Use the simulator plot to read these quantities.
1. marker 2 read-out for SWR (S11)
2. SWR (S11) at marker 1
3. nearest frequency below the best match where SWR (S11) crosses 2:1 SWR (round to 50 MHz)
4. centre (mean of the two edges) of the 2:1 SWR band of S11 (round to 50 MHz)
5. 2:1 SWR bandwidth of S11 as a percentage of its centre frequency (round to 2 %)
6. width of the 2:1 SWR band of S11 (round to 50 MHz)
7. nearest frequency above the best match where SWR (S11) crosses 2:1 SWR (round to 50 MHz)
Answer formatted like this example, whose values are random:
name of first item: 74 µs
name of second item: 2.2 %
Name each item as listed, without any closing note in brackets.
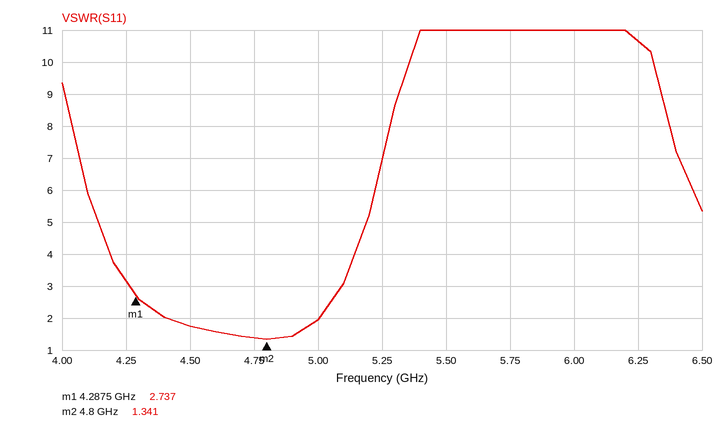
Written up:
marker 2 read-out for SWR: 1.341
SWR (S11) at marker 1: 2.737
nearest frequency below the best match where SWR (S11) crosses 2:1 SWR: 4.40 GHz
centre (mean of the two edges) of the 2:1 SWR band of S11: 4.70 GHz
2:1 SWR bandwidth of S11 as a percentage of its centre frequency: 12 %
width of the 2:1 SWR band of S11: 600 MHz
nearest frequency above the best match where SWR (S11) crosses 2:1 SWR: 5.00 GHz
